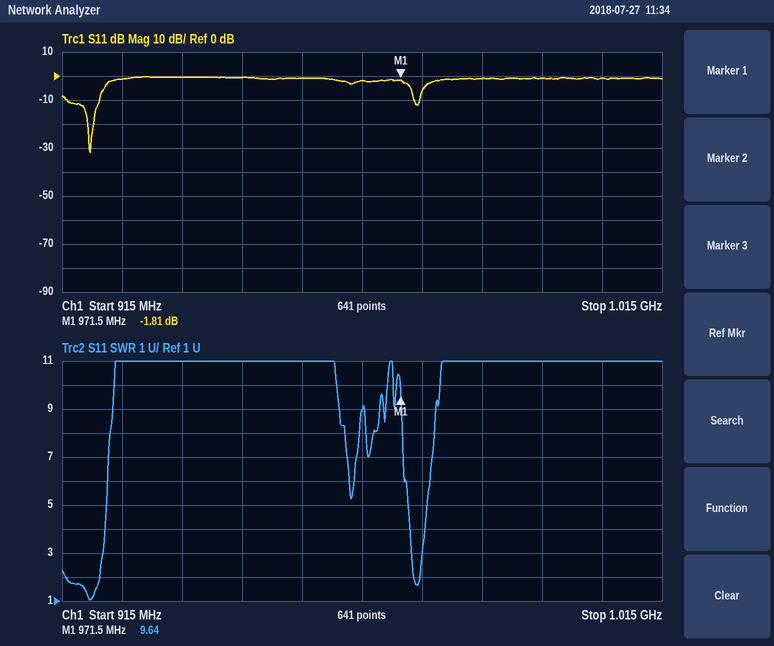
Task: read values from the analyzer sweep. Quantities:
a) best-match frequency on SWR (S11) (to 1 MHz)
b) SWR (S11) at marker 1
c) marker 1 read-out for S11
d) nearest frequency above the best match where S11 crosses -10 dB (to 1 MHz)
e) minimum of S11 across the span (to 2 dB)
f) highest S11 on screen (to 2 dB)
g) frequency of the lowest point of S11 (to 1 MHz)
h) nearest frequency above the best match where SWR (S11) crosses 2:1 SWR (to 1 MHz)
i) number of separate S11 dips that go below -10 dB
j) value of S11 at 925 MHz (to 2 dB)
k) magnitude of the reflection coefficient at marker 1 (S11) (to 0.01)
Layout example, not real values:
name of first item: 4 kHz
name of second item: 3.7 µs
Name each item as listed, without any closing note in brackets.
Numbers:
best-match frequency on SWR (S11): 920 MHz
SWR (S11) at marker 1: 9.64
marker 1 read-out for S11: -1.81 dB
nearest frequency above the best match where S11 crosses -10 dB: 921 MHz
minimum of S11 across the span: -32 dB
highest S11 on screen: 0 dB
frequency of the lowest point of S11: 920 MHz
nearest frequency above the best match where SWR (S11) crosses 2:1 SWR: 921 MHz
number of separate S11 dips that go below -10 dB: 2
value of S11 at 925 MHz: -2 dB
magnitude of the reflection coefficient at marker 1 (S11): 0.81
